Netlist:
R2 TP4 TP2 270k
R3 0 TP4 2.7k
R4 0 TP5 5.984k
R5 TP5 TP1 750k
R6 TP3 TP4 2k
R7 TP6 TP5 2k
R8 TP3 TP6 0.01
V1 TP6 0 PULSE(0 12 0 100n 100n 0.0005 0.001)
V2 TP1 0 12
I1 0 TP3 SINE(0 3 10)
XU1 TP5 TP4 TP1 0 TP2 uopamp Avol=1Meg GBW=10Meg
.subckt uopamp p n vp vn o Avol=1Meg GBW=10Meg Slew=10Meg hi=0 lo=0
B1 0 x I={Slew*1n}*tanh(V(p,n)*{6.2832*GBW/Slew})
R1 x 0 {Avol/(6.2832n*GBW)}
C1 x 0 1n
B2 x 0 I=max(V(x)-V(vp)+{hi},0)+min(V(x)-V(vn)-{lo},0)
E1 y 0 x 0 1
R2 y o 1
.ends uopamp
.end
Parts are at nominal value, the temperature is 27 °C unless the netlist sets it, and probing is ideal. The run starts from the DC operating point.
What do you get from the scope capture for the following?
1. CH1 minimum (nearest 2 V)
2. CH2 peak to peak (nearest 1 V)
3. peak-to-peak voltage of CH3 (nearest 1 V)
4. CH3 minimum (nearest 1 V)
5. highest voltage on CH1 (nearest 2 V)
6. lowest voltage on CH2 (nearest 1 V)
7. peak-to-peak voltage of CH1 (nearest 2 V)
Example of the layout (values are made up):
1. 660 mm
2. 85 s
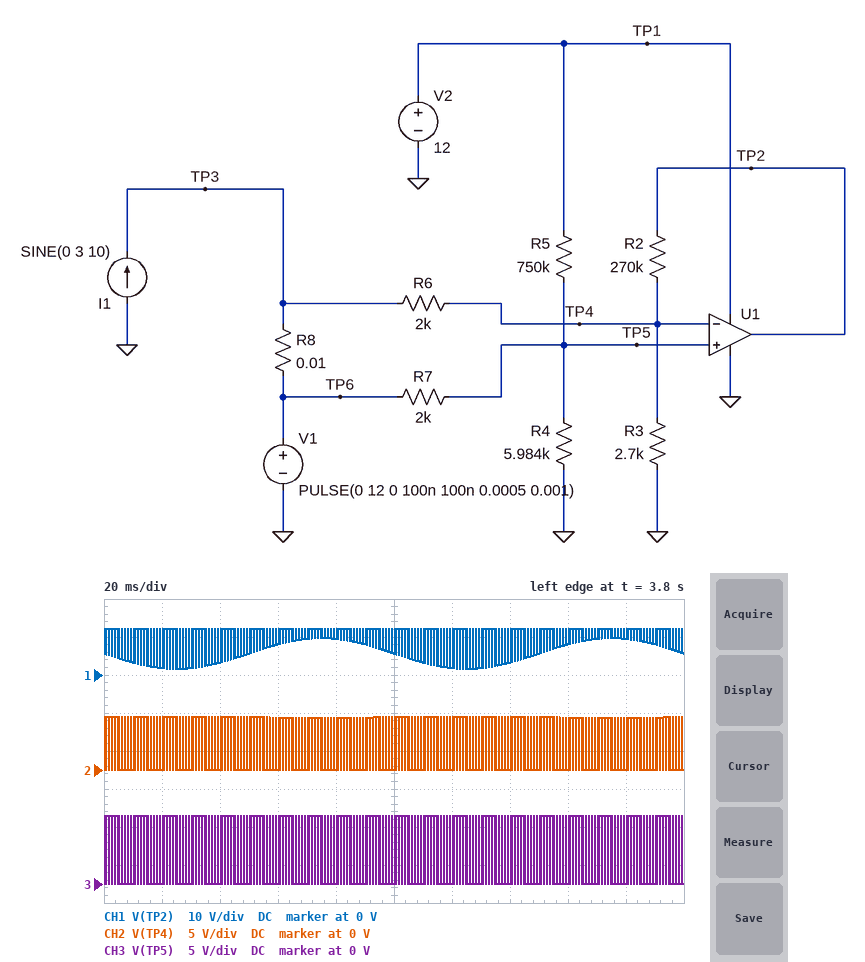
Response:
1. 2 V
2. 7 V
3. 9 V
4. 0 V
5. 12 V
6. 0 V
7. 10 V
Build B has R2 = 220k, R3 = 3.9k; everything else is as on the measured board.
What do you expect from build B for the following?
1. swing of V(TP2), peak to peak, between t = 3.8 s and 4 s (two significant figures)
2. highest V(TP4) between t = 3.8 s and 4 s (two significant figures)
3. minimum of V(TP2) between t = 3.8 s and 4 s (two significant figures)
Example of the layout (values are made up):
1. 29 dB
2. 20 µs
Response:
1. 11 V
2. 8.0 V
3. 710 mV
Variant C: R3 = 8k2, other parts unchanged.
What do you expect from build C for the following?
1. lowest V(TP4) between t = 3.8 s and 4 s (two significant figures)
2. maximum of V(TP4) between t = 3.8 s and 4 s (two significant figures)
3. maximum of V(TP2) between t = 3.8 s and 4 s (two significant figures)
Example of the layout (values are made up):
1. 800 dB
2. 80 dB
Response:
1. -24 mV
2. 9.6 V
3. 8.1 V
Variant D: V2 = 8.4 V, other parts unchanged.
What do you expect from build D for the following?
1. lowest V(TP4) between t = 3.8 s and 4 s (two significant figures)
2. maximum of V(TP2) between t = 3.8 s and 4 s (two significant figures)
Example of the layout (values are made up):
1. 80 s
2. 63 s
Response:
1. 17 mV
2. 8.4 V
